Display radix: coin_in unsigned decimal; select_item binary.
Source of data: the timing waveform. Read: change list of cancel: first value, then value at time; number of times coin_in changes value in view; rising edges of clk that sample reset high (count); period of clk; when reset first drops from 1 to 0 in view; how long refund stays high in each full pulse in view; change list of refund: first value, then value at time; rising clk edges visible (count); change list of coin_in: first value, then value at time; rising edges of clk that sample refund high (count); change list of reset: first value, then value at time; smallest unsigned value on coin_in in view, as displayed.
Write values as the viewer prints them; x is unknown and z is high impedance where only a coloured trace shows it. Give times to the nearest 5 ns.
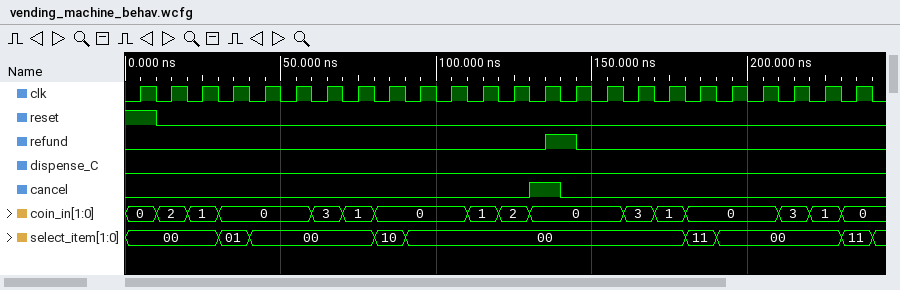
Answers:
0, 1 at 130 ns, 0 at 140 ns
15
1
10 ns
10 ns
10 ns
0, 1 at 135 ns, 0 at 145 ns
24
0, 2 at 10 ns, 1 at 20 ns, 0 at 30 ns, 3 at 60 ns, 1 at 70 ns, 0 at 80 ns, 1 at 110 ns, 2 at 120 ns, 0 at 130 ns, 3 at 160 ns, 1 at 170 ns, 0 at 180 ns, 3 at 210 ns, 1 at 220 ns, 0 at 230 ns
1
1, 0 at 10 ns
0
